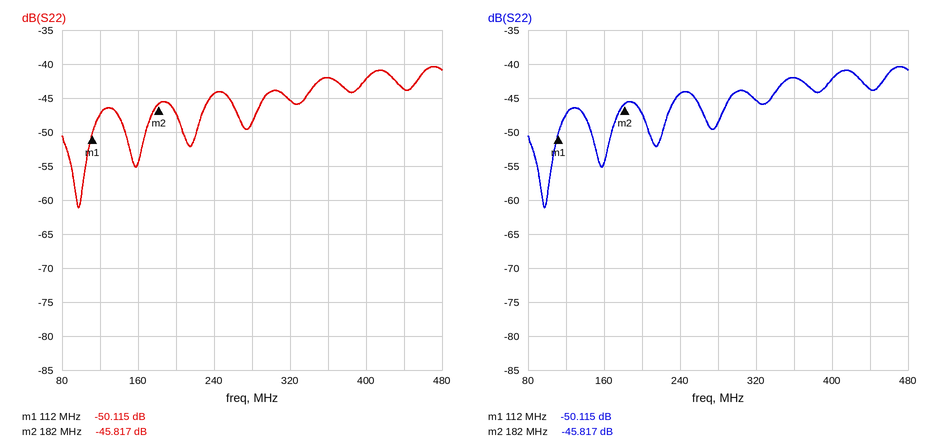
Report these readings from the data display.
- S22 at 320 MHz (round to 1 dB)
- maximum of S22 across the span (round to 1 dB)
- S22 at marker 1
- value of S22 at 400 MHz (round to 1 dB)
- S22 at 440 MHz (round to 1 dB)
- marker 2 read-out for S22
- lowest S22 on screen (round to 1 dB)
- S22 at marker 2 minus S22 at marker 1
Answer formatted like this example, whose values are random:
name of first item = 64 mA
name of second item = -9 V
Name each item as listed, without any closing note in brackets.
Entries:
S22 at 320 MHz = -45 dB
maximum of S22 across the span = -40 dB
S22 at marker 1 = -50.115 dB
value of S22 at 400 MHz = -42 dB
S22 at 440 MHz = -44 dB
marker 2 read-out for S22 = -45.817 dB
lowest S22 on screen = -61 dB
S22 at marker 2 minus S22 at marker 1 = 4.298 dB
